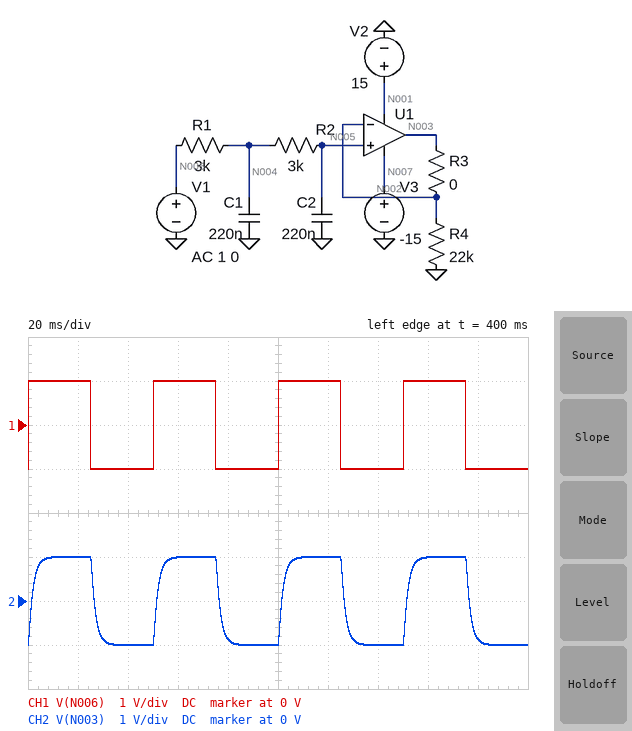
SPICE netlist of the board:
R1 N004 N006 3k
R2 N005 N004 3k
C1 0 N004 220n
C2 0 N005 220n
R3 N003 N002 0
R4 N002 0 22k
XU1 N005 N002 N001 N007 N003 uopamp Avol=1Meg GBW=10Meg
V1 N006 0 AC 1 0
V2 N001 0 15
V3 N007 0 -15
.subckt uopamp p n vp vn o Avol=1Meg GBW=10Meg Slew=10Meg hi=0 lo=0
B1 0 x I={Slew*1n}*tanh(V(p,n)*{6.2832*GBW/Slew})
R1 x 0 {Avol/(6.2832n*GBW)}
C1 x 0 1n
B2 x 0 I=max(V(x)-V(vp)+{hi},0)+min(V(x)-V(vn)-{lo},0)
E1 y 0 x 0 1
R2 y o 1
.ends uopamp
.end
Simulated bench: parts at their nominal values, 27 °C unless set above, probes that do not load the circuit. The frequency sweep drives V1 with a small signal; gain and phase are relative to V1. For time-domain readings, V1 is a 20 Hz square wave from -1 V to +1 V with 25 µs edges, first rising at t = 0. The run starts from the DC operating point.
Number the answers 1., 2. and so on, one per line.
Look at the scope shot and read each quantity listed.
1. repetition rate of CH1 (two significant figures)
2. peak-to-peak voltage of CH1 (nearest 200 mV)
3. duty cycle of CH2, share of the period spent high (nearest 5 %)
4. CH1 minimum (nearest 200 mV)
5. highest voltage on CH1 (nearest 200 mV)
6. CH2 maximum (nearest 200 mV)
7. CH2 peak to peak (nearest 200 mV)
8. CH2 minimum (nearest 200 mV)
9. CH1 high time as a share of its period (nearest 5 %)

1. 20 Hz
2. 2.0 V
3. 50 %
4. -1.0 V
5. 1.0 V
6. 1.0 V
7. 2.0 V
8. -1.0 V
9. 50 %
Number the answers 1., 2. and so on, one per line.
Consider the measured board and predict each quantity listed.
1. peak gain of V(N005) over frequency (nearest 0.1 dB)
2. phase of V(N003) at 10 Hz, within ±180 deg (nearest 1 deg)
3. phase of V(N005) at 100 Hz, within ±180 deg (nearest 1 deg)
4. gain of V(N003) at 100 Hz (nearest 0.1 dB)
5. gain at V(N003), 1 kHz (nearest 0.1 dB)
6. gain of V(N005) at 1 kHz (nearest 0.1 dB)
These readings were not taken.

1. 0 dB
2. -7 deg
3. -56 deg
4. -3.5 dB
5. -26.2 dB
6. -26.2 dB
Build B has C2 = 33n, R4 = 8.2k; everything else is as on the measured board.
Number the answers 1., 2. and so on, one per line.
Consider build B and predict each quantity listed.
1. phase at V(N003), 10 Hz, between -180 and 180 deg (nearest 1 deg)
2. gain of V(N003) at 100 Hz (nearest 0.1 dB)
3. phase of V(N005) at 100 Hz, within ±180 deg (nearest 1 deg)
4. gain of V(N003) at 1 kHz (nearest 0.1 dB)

1. -3 deg
2. -0.9 dB
3. -29 deg
4. -15.0 dB
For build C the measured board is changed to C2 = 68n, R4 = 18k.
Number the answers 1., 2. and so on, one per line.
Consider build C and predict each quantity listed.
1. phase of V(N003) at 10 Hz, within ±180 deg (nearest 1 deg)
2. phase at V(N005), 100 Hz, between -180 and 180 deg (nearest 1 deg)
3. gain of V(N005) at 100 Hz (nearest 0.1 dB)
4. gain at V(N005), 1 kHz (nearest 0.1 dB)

1. -4 deg
2. -35 deg
3. -1.3 dB
4. -18.0 dB
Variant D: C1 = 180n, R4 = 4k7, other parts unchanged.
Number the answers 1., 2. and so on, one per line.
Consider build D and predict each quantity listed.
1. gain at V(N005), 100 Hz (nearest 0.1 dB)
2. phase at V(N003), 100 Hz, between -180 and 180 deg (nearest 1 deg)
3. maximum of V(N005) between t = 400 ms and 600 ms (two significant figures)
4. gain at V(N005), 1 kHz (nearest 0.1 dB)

1. -3.2 dB
2. -54 deg
3. 1.0 V
4. -24.9 dB
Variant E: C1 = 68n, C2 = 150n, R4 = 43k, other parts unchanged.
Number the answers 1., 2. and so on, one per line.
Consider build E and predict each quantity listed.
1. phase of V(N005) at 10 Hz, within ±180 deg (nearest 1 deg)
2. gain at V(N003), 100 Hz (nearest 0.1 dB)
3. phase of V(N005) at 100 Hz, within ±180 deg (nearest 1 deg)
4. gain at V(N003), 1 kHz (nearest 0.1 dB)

1. -4 deg
2. -1.5 dB
3. -36 deg
4. -17.4 dB
